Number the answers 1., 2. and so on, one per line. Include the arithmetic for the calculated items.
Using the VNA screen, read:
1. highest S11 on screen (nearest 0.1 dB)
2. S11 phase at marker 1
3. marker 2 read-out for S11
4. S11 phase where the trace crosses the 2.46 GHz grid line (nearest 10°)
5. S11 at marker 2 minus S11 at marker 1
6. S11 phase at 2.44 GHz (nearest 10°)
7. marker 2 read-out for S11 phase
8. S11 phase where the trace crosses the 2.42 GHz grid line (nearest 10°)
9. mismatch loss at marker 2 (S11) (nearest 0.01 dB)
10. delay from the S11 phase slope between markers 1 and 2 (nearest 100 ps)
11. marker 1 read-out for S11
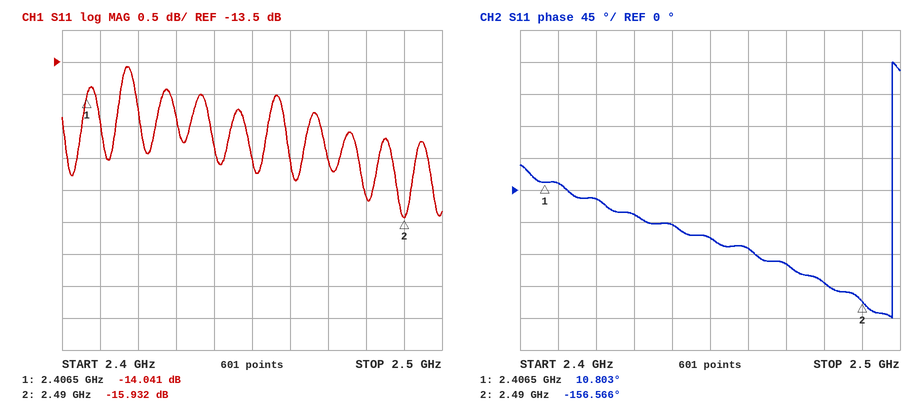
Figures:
1. -13.6 dB
2. 10.803°
3. -15.932 dB
4. -80°
5. -15.932 − (-14.041) = -1.891 dB
6. -50°
7. -156.566°
8. -10°
9. −10 log10(1 − 10^(-15.932/10)) ≈ 0.11 dB
10. −(-156.566° − (10.803°))/(360° × 83.5 MHz) ≈ 5.6 ns
11. -14.041 dB
